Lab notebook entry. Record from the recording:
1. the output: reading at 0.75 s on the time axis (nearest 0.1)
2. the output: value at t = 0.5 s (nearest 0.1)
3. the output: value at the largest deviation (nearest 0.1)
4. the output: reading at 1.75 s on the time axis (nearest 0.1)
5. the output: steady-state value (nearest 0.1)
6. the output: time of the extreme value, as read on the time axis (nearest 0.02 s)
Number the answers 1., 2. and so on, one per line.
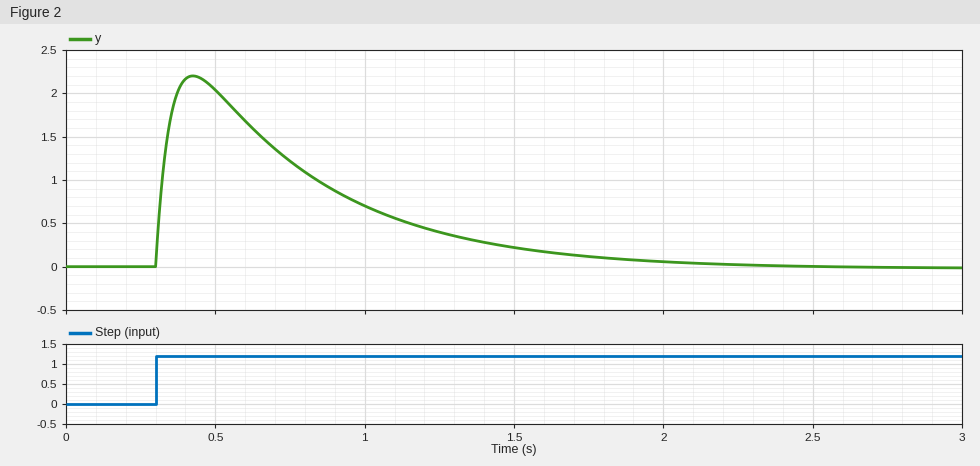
1. 1.2
2. 2.0
3. 2.2
4. 0.1
5. 0.0
6. 0.42 s
